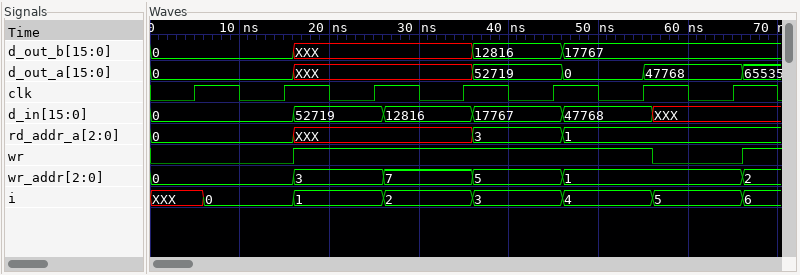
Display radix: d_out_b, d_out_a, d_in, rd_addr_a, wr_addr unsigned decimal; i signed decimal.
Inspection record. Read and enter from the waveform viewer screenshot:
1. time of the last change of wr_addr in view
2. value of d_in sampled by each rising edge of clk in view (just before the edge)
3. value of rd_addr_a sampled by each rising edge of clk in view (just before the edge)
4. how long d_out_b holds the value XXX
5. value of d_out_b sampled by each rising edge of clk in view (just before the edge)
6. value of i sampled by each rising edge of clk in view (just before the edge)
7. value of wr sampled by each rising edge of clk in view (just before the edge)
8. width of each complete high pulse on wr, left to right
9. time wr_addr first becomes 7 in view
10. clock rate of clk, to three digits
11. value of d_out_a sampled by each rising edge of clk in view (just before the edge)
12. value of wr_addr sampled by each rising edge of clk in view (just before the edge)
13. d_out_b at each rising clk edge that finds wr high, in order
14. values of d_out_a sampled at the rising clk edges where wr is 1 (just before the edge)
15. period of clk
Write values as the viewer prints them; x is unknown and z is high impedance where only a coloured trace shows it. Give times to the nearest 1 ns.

66 ns
0, 0, 52719, 12816, 17767, 47768, XXX
0, 0, XXX, XXX, 3, 1, 1
20 ns
0, 0, XXX, XXX, 12816, 17767, 17767
XXX, 0, 1, 2, 3, 4, 5
0 0 1 1 1 1 0
40 ns
26 ns
100 MHz
0, 0, XXX, XXX, 52719, 0, 47768
0, 0, 3, 7, 5, 1, 1
XXX, XXX, 12816, 17767
XXX, XXX, 52719, 0
10 ns
